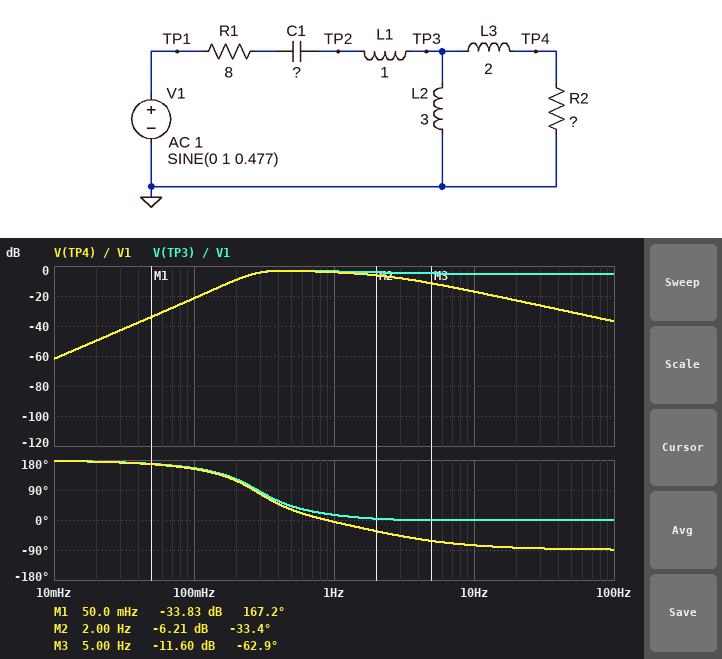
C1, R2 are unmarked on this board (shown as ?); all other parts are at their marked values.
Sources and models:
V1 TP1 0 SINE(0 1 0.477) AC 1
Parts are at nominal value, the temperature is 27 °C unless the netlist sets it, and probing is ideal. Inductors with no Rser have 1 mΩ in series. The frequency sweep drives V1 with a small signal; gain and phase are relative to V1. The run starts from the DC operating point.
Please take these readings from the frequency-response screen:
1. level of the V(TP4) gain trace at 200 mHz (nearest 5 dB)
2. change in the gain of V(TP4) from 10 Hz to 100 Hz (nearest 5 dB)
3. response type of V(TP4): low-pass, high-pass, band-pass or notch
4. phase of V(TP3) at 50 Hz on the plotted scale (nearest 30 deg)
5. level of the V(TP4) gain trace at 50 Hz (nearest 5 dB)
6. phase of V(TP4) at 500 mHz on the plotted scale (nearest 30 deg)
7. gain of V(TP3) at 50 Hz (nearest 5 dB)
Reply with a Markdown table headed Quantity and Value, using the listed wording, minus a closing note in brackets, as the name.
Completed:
| Quantity | Value |
|---|---|
| level of the V(TP4) gain trace at 200 mHz | -10 dB |
| change in the gain of V(TP4) from 10 Hz to 100 Hz | -20 dB |
| response type of V(TP4): low-pass, high-pass, band-pass or notch | band-pass |
| phase of V(TP3) at 50 Hz on the plotted scale | 0 deg |
| level of the V(TP4) gain trace at 50 Hz | -30 dB |
| phase of V(TP4) at 500 mHz on the plotted scale | 30 deg |
| gain of V(TP3) at 50 Hz | -5 dB |
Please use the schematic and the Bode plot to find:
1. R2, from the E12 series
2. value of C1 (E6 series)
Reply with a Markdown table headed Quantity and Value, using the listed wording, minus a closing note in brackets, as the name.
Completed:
| Quantity | Value |
|---|---|
| R2, from the E12 series | 33 Ω |
| value of C1 | 68 mF |
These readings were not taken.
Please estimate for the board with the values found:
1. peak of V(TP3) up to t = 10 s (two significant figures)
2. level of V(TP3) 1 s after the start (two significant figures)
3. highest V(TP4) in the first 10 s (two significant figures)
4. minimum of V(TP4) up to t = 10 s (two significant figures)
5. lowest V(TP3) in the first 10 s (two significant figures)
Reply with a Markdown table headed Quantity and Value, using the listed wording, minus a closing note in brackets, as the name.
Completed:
| Quantity | Value |
|---|---|
| peak of V(TP3) up to t = 10 s | 750 mV |
| level of V(TP3) 1 s after the start | -440 mV |
| highest V(TP4) in the first 10 s | 740 mV |
| minimum of V(TP4) up to t = 10 s | -700 mV |
| lowest V(TP3) in the first 10 s | -710 mV |
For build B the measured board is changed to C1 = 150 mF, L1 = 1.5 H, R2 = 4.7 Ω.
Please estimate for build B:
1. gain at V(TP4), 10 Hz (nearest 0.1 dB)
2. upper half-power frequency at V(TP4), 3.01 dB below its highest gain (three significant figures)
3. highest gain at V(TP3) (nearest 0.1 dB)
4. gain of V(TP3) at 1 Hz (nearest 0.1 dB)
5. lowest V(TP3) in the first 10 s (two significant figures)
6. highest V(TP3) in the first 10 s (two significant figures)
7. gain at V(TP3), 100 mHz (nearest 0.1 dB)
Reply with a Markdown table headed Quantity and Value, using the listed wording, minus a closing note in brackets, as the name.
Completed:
| Quantity | Value |
|---|---|
| gain at V(TP4), 10 Hz | -35.6 dB |
| upper half-power frequency at V(TP4), 3.01 dB below its highest gain | 734 mHz |
| highest gain at V(TP3) | -7.0 dB |
| gain of V(TP3) at 1 Hz | -7.5 dB |
| lowest V(TP3) in the first 10 s | -400 mV |
| highest V(TP3) in the first 10 s | 390 mV |
| gain at V(TP3), 100 mHz | -17.2 dB |
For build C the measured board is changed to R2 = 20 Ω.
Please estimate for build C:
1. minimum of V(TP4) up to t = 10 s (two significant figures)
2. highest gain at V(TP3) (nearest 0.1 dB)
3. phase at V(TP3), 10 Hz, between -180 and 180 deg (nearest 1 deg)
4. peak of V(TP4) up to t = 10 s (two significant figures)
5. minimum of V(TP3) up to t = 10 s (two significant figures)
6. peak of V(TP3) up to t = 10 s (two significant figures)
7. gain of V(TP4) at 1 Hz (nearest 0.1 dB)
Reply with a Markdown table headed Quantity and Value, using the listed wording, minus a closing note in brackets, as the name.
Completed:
| Quantity | Value |
|---|---|
| minimum of V(TP4) up to t = 10 s | -610 mV |
| highest gain at V(TP3) | -3.9 dB |
| phase at V(TP3), 10 Hz, between -180 and 180 deg | 1 deg |
| peak of V(TP4) up to t = 10 s | 650 mV |
| minimum of V(TP3) up to t = 10 s | -640 mV |
| peak of V(TP3) up to t = 10 s | 680 mV |
| gain of V(TP4) at 1 Hz | -5.8 dB |
